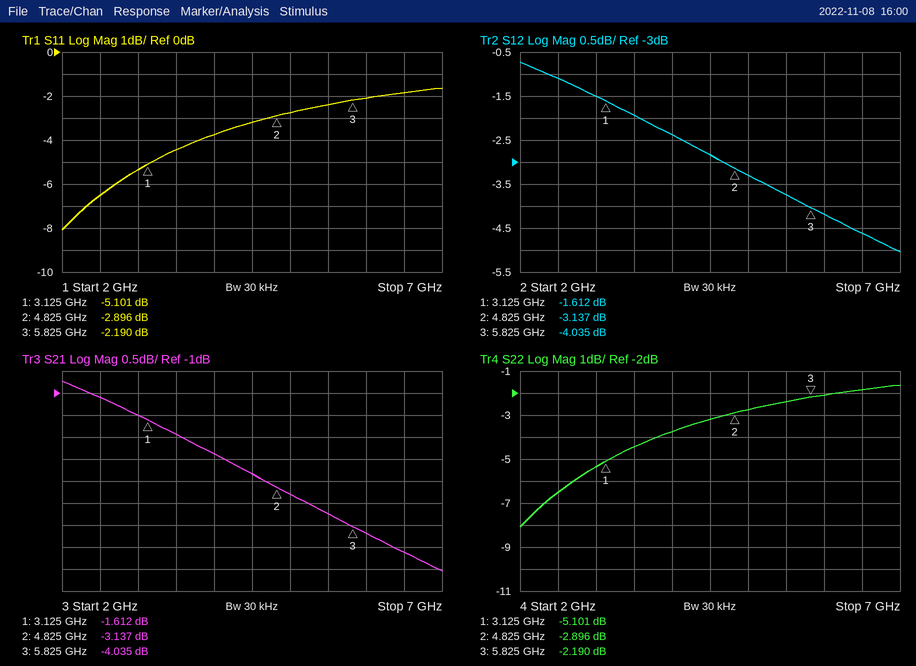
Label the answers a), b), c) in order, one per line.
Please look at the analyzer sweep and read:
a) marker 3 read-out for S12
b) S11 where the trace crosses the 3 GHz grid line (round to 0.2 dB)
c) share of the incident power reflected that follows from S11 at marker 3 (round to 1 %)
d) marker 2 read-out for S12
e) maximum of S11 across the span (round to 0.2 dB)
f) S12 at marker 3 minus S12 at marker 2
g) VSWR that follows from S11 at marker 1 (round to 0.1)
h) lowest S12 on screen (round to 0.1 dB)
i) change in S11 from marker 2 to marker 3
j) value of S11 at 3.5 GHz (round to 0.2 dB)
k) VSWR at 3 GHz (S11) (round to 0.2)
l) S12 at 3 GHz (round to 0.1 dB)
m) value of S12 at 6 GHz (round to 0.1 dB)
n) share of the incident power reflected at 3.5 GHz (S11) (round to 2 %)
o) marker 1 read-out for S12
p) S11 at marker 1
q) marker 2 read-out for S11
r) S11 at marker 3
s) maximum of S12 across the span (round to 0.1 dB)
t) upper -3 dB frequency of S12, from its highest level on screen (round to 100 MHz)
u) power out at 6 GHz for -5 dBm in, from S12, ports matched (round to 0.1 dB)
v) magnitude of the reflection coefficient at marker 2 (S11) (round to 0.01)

a) -4.035 dB
b) -5.4 dB
c) 60 %
d) -3.137 dB
e) -1.6 dB
f) -0.898 dB
g) 3.5
h) -5.0 dB
i) 0.706 dB
j) -4.4 dB
k) 3.4
l) -1.5 dB
m) -4.2 dB
n) 36 %
o) -1.612 dB
p) -5.101 dB
q) -2.896 dB
r) -2.190 dB
s) -0.7 dB
t) 5.5 GHz
u) -9.2 dBm
v) 0.72
